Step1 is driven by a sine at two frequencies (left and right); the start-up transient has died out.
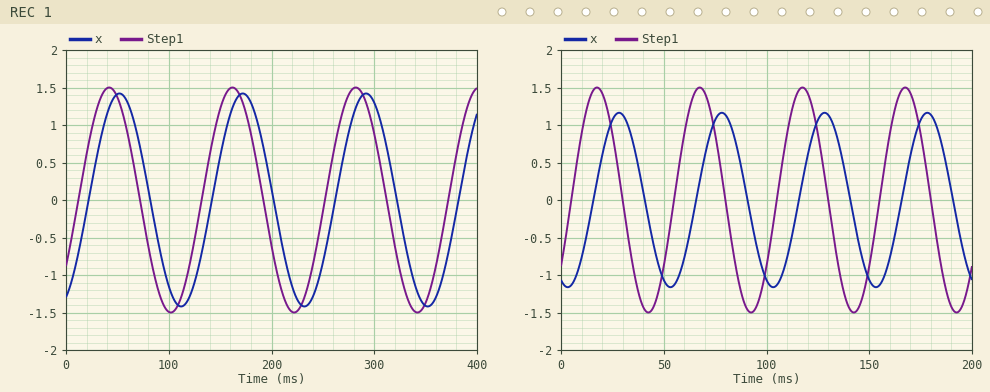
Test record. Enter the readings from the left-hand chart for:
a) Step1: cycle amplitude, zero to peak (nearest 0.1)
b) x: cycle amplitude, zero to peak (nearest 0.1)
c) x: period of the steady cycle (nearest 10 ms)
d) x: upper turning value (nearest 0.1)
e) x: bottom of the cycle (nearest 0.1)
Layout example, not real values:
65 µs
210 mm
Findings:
1.5
1.4
120 ms
1.4
-1.4
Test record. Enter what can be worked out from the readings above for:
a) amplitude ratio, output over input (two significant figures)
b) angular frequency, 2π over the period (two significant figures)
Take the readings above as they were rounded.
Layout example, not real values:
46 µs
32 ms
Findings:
0.93
0.052 rad/ms
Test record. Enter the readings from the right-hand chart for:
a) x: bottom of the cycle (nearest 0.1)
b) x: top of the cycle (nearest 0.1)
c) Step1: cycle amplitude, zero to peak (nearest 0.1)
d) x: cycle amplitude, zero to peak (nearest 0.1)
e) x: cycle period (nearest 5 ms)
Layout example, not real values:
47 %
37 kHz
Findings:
-1.2
1.2
1.5
1.2
50 ms
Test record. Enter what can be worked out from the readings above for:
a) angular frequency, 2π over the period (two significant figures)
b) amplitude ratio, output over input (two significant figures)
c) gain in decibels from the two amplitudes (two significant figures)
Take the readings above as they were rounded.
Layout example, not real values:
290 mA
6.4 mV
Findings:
0.13 rad/ms
0.80
-1.9 dB
